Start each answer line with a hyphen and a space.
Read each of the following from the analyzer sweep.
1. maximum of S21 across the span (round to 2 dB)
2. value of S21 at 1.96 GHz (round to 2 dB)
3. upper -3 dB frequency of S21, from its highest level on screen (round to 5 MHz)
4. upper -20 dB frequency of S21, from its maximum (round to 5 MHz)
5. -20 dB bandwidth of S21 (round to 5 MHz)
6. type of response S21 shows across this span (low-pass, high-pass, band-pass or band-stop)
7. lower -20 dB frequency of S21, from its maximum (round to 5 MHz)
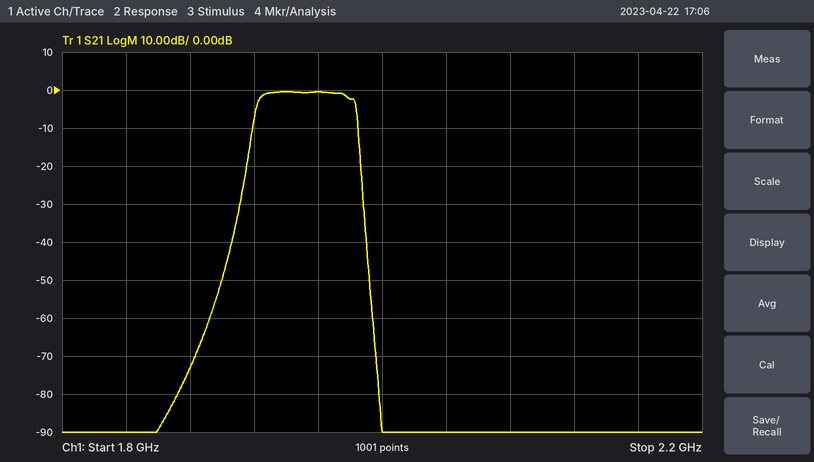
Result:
- 0 dB
- 0 dB
- 1.985 GHz
- 1.985 GHz
- 70 MHz
- band-pass
- 1.915 GHz
